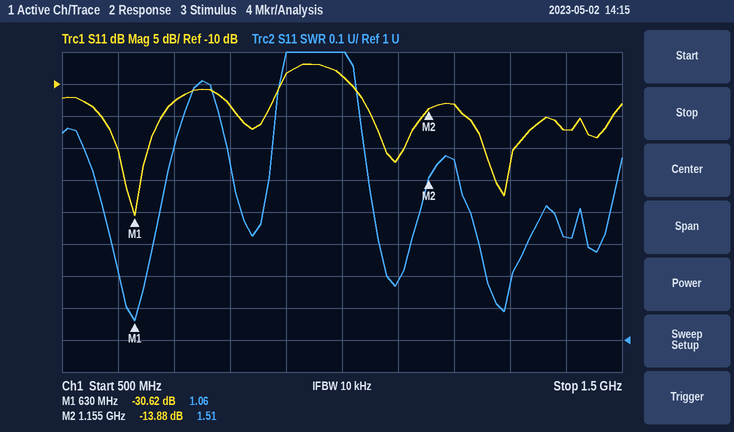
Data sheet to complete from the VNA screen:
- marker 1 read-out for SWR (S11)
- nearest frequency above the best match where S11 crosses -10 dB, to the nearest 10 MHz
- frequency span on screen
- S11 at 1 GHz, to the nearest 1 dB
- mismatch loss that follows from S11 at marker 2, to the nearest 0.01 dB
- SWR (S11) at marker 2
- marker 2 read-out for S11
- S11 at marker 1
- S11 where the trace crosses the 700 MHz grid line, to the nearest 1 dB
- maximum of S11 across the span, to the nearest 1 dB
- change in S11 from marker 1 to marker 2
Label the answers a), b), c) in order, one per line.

a) 1.06
b) 890 MHz
c) 1 GHz
d) -9 dB
e) 0.18 dB
f) 1.51
g) -13.88 dB
h) -30.62 dB
i) -13 dB
j) -7 dB
k) 16.74 dB
